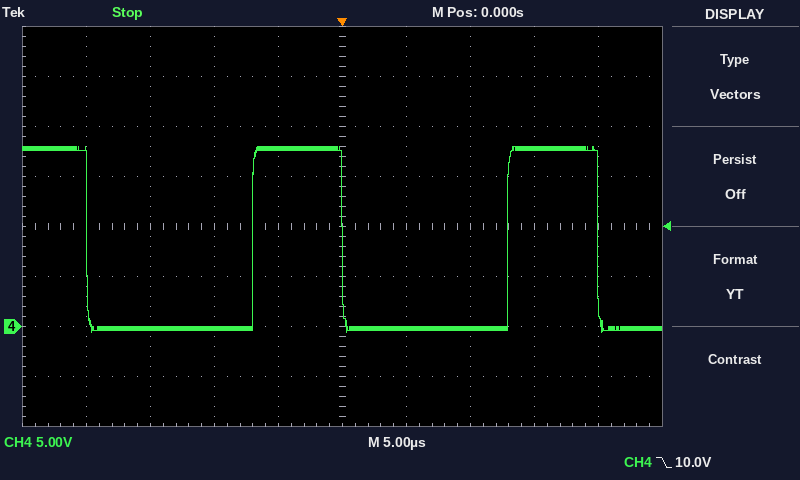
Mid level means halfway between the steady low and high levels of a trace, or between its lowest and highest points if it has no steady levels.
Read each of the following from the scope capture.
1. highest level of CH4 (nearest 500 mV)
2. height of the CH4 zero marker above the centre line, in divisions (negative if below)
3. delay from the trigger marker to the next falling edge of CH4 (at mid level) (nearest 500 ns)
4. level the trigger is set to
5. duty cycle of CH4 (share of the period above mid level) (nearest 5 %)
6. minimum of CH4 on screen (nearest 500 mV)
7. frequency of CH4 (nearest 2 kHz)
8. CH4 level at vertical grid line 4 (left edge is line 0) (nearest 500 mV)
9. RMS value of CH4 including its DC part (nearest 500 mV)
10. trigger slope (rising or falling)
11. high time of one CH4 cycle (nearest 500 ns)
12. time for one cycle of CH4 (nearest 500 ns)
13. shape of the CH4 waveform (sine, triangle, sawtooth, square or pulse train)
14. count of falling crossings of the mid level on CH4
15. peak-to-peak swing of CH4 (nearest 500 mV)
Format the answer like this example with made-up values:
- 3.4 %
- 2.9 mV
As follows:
- 18.0 V
- -2.0 div
- 20.0 µs
- 10.0 V
- 35 %
- -500 mV
- 50 kHz
- 18.0 V
- 10.5 V
- falling
- 7.0 µs
- 20.0 µs
- pulse train
- 3
- 18.5 V
